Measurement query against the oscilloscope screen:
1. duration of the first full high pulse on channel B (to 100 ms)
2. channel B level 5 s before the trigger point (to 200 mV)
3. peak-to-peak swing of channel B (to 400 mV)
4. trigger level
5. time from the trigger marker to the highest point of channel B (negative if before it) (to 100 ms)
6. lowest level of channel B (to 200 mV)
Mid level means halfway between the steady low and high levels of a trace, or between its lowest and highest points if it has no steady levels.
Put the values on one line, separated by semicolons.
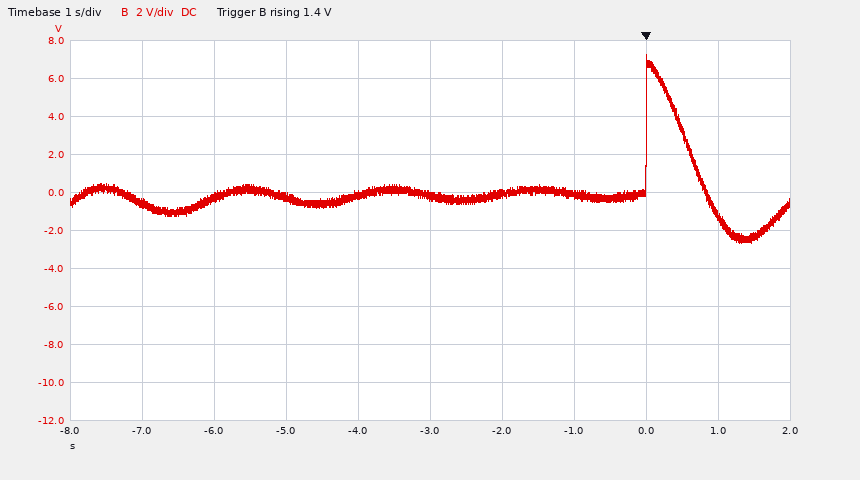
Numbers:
600 ms; -200 mV; 10.0 V; 1.4 V; 0.0 s; -2.6 V
